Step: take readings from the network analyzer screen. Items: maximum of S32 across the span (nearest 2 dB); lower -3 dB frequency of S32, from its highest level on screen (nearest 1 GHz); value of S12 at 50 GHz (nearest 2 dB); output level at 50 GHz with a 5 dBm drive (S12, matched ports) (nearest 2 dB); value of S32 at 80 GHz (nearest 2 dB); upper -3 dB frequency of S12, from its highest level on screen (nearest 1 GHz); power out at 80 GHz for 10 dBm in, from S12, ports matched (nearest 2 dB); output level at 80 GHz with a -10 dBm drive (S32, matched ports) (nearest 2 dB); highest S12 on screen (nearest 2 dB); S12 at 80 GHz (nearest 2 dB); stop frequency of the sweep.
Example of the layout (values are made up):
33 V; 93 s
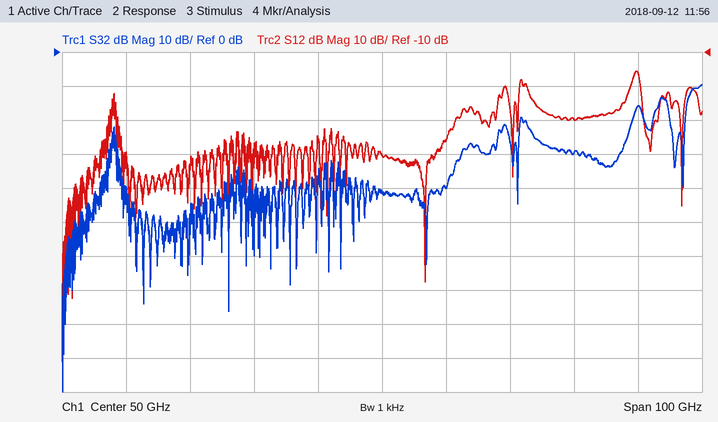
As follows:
-10 dB; 98 GHz; -40 dB; -36 dBm; -30 dB; 90 GHz; -20 dBm; -40 dBm; -16 dB; -30 dB; 100 GHz
